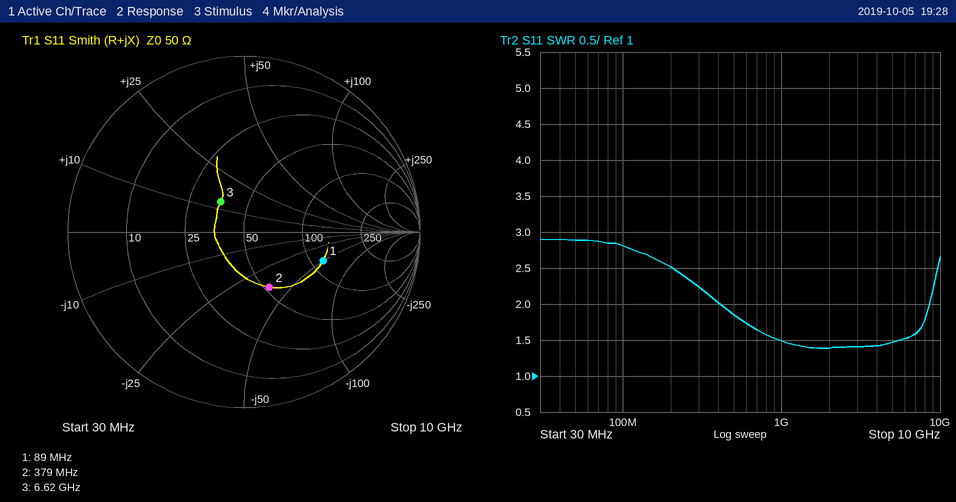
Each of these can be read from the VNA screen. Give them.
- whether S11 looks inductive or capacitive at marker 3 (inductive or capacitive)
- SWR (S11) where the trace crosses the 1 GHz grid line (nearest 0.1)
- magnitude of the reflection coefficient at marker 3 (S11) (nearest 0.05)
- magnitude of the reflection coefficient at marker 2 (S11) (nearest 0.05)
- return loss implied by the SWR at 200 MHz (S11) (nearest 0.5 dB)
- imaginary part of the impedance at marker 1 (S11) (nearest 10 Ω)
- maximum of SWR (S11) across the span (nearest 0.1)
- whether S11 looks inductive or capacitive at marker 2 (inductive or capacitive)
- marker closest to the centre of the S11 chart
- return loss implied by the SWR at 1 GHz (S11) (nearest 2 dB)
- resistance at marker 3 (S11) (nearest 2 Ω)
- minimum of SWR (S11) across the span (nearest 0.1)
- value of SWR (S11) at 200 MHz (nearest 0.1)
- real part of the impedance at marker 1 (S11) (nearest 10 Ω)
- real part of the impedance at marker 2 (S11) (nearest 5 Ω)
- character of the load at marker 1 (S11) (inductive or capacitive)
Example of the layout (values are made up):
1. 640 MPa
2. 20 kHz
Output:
1. inductive
2. 1.5
3. 0.20
4. 0.35
5. 7.5 dB
6. -50 Ω
7. 2.9
8. capacitive
9. marker 3
10. 14 dB
11. 36 Ω
12. 1.4
13. 2.5
14. 120 Ω
15. 55 Ω
16. capacitive
